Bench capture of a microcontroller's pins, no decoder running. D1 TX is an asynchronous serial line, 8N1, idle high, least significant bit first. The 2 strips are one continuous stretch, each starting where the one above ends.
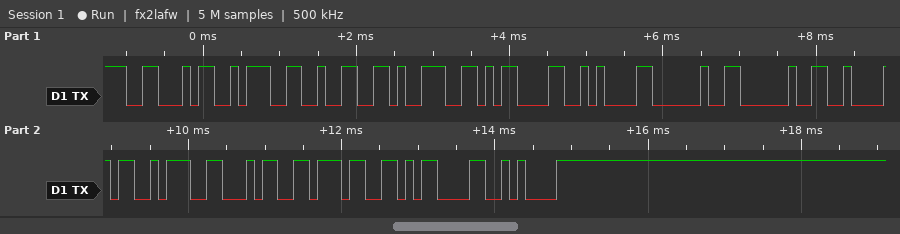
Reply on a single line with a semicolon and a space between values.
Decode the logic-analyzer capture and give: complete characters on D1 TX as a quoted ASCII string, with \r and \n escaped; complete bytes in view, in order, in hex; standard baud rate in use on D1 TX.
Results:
"F:29\r\n  B:47\r\n"; 46 3A 32 39 0D 0A 20 20 42 3A 34 37 0D 0A; 9600 baud
